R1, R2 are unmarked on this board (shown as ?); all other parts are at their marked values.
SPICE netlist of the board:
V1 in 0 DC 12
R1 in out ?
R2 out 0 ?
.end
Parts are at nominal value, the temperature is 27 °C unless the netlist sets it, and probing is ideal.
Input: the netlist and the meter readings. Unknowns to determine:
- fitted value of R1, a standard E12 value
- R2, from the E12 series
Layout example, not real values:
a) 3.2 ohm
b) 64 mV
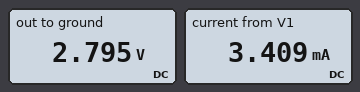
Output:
a) 2.7 kΩ
b) 820 Ω
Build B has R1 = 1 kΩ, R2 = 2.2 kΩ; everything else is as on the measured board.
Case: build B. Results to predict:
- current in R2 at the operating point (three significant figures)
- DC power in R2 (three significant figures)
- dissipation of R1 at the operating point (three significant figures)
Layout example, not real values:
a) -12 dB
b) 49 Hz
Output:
a) 3.75 mA
b) 30.9 mW
c) 14.1 mW
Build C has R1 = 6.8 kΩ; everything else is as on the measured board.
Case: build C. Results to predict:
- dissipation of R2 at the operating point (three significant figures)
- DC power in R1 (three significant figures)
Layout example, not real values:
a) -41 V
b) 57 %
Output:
a) 2.03 mW
b) 16.9 mW
